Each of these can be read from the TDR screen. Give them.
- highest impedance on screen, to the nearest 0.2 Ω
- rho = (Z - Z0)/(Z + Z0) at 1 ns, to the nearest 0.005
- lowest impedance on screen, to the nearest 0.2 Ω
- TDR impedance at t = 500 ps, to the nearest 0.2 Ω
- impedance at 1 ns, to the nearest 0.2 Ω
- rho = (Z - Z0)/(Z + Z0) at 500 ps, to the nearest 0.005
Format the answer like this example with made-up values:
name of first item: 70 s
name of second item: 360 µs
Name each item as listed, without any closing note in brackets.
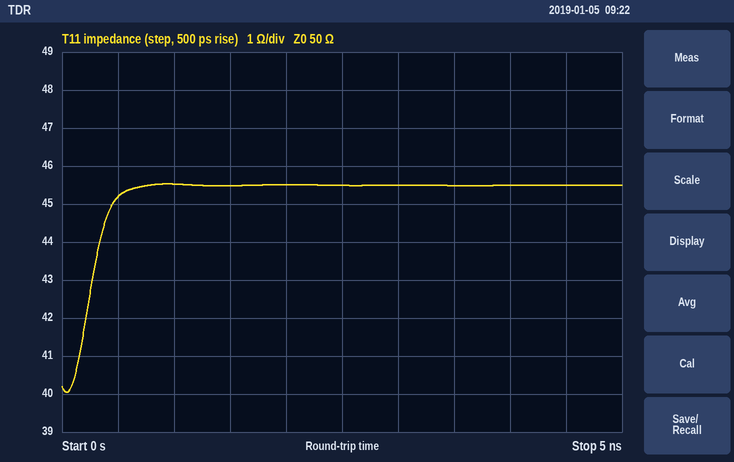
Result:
highest impedance on screen, to the nearest 0.2 Ω: 45.6 Ω
rho = (Z - Z0)/(Z + Z0) at 1 ns, to the nearest 0.005: -0.045
lowest impedance on screen, to the nearest 0.2 Ω: 40.0 Ω
TDR impedance at t = 500 ps, to the nearest 0.2 Ω: 45.2 Ω
impedance at 1 ns, to the nearest 0.2 Ω: 45.6 Ω
rho = (Z - Z0)/(Z + Z0) at 500 ps, to the nearest 0.005: -0.050
